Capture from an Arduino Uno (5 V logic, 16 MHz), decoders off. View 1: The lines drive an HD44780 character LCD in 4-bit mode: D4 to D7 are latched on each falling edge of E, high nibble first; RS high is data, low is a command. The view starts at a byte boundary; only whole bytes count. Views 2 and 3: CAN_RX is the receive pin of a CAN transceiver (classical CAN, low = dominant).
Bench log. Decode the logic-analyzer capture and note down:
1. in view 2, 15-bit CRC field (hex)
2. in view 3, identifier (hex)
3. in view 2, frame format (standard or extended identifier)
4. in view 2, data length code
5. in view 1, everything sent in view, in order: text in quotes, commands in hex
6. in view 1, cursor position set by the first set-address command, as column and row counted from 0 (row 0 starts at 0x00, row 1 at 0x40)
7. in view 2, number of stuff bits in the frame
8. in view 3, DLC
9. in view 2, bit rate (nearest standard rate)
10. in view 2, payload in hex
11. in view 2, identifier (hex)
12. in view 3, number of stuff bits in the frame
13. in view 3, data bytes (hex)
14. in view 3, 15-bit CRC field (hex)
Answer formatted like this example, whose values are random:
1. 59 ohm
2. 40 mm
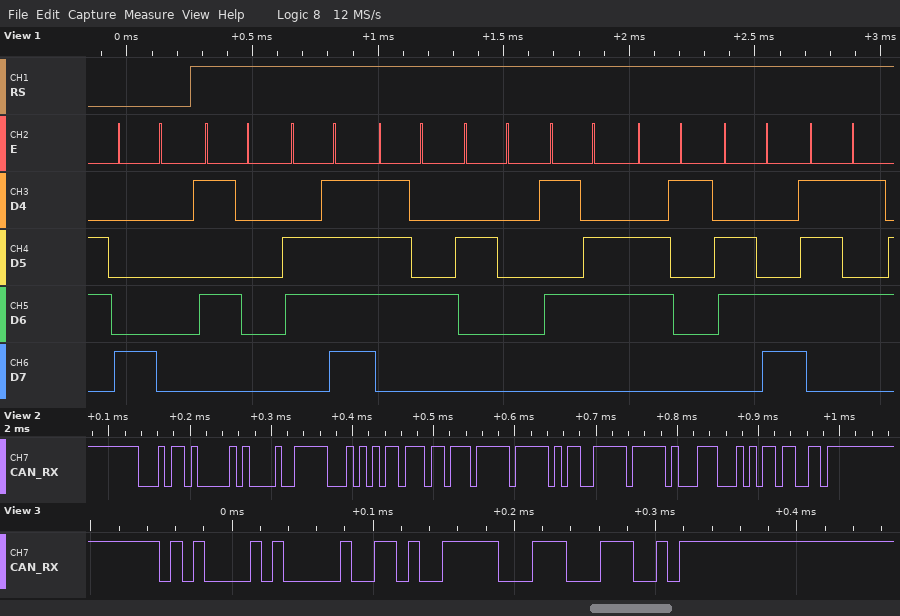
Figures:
1. 0x0AD9
2. 0x50A
3. standard
4. 8
5. 0x80 "Pot Valu"
6. column 0, row 0
7. 6
8. 1
9. 125 kbit/s
10. 4F 95 6E DD FF D9 FF C7
11. 0x168
12. 2
13. A7
14. 0x671C
